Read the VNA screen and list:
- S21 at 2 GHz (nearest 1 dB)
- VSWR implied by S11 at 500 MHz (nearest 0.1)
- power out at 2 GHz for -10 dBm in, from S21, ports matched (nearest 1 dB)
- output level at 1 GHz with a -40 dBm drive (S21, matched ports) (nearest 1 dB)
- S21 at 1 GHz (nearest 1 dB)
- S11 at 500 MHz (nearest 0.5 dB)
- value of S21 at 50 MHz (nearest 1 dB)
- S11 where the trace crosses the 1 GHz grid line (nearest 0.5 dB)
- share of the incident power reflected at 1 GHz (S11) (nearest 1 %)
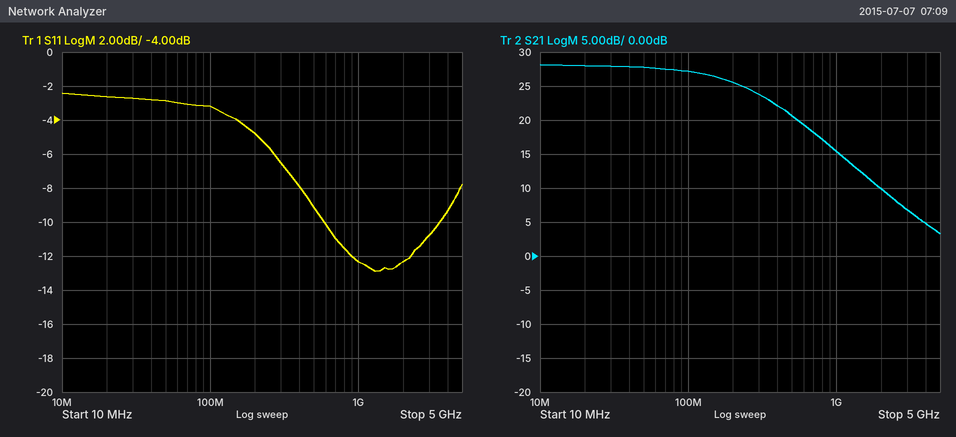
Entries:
10 dB
2.1
0 dBm
-25 dBm
15 dB
-9.0 dB
28 dB
-12.5 dB
6 %
